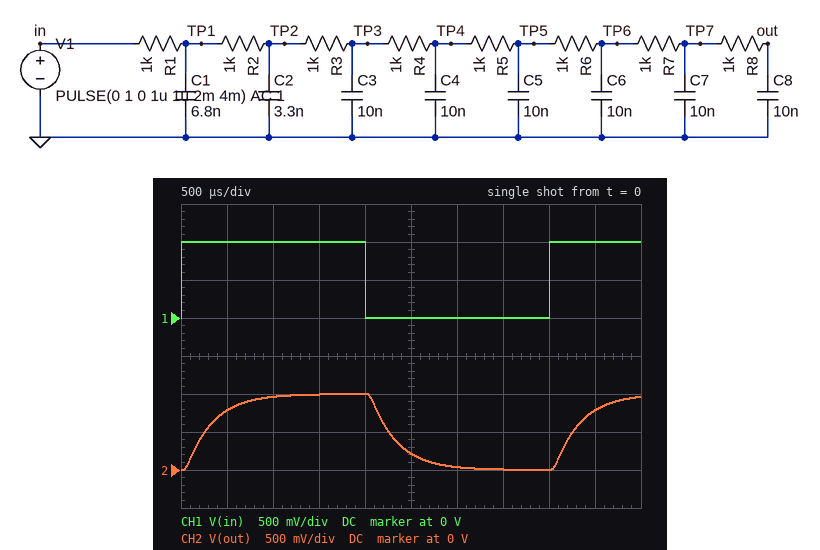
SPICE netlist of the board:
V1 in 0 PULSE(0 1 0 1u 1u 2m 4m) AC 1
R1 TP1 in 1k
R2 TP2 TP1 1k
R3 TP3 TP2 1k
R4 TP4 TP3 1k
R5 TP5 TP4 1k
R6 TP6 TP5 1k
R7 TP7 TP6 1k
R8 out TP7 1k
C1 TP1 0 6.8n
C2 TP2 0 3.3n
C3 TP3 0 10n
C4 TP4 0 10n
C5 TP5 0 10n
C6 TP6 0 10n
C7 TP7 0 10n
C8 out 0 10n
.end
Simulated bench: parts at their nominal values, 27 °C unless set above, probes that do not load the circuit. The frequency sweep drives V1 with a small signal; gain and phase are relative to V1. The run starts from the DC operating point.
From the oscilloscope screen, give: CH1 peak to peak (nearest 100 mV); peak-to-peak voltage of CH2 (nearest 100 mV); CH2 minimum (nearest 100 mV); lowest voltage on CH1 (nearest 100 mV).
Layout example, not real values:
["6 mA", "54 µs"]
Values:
["1.0 V", "1.0 V", "0 V", "0 V"]
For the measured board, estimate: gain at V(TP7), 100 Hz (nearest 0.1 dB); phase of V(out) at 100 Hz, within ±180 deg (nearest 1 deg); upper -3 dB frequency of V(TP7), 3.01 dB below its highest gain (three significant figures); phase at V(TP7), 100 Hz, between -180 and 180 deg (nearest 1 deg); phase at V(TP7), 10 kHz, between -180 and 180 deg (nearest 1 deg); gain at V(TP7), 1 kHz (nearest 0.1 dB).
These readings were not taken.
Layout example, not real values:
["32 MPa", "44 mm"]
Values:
["-0.1 dB", "-12 deg", "548 Hz", "-12 deg", "152 deg", "-6.4 dB"]
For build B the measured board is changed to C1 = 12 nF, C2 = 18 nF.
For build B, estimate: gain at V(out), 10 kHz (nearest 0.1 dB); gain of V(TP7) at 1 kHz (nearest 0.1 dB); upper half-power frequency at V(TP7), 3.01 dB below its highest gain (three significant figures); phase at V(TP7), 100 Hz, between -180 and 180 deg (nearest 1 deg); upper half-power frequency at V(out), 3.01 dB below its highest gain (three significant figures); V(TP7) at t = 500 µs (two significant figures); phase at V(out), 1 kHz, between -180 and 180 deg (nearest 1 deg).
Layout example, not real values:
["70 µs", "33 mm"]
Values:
["-38.6 dB", "-6.9 dB", "518 Hz", "-13 deg", "517 Hz", "760 mV", "-89 deg"]
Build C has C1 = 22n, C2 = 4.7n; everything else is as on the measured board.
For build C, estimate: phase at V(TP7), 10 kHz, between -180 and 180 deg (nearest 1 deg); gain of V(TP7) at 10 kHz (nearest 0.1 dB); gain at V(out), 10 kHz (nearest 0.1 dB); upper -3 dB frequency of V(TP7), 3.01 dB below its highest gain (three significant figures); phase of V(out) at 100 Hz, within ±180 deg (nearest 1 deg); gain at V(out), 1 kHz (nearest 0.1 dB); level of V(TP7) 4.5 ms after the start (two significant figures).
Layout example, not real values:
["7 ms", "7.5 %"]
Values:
["124 deg", "-35.8 dB", "-37.2 dB", "537 Hz", "-13 deg", "-6.6 dB", "780 mV"]
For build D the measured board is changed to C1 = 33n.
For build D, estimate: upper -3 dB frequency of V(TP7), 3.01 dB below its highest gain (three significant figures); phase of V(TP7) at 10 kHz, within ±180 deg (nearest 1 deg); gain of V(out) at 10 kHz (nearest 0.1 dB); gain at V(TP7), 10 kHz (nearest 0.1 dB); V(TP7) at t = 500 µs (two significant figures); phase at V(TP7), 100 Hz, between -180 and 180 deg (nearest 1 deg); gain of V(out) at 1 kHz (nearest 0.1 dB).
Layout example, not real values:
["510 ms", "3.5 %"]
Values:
["532 Hz", "117 deg", "-38.9 dB", "-37.5 dB", "770 mV", "-13 deg", "-6.7 dB"]
